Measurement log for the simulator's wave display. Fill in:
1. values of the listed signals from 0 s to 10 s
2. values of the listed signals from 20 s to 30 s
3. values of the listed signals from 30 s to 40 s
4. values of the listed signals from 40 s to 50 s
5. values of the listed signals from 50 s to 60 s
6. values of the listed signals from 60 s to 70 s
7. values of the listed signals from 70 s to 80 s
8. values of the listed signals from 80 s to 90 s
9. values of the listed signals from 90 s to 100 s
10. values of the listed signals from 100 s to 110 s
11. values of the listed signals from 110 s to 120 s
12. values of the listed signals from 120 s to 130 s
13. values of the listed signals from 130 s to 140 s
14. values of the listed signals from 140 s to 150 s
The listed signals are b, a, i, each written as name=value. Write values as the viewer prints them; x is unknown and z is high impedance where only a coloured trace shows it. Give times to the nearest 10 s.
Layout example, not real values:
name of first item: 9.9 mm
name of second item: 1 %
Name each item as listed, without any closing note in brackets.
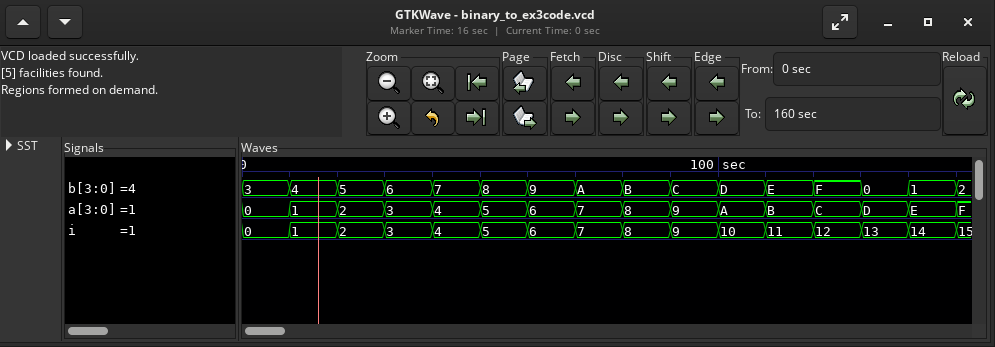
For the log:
values of the listed signals from 0 s to 10 s: b=3, a=0, i=0
values of the listed signals from 20 s to 30 s: b=5, a=2, i=2
values of the listed signals from 30 s to 40 s: b=6, a=3, i=3
values of the listed signals from 40 s to 50 s: b=7, a=4, i=4
values of the listed signals from 50 s to 60 s: b=8, a=5, i=5
values of the listed signals from 60 s to 70 s: b=9, a=6, i=6
values of the listed signals from 70 s to 80 s: b=A, a=7, i=7
values of the listed signals from 80 s to 90 s: b=B, a=8, i=8
values of the listed signals from 90 s to 100 s: b=C, a=9, i=9
values of the listed signals from 100 s to 110 s: b=D, a=A, i=10
values of the listed signals from 110 s to 120 s: b=E, a=B, i=11
values of the listed signals from 120 s to 130 s: b=F, a=C, i=12
values of the listed signals from 130 s to 140 s: b=0, a=D, i=13
values of the listed signals from 140 s to 150 s: b=1, a=E, i=14
